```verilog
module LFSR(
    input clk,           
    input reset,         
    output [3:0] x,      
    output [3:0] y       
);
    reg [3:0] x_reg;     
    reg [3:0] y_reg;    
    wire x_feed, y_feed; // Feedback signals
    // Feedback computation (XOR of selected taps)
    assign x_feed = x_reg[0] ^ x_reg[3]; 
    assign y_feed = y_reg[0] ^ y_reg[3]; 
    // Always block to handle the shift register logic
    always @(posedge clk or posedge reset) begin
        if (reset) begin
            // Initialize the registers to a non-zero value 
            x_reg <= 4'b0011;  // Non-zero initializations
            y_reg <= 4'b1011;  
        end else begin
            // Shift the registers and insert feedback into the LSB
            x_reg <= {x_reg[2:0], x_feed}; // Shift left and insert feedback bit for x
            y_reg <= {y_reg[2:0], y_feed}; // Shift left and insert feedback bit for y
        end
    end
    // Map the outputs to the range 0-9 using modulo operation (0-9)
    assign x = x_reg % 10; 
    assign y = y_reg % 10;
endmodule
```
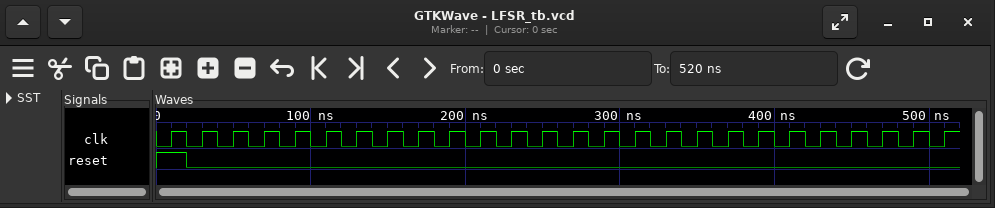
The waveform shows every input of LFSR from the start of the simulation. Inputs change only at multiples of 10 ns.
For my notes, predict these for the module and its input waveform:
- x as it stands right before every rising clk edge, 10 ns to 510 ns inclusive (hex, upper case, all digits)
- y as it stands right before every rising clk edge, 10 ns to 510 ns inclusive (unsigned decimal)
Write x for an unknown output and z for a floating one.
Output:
3, 3, 7, 5, 4, 3, 0, 5, 1, 6, 2, 9, 2, 4, 8, 1, 3, 7, 5, 4, 3, 0, 5, 1, 6, 2
1, 1, 6, 2, 9, 2, 4, 8, 1, 3, 7, 5, 4, 3, 0, 5, 1, 6, 2, 9, 2, 4, 8, 1, 3, 7
